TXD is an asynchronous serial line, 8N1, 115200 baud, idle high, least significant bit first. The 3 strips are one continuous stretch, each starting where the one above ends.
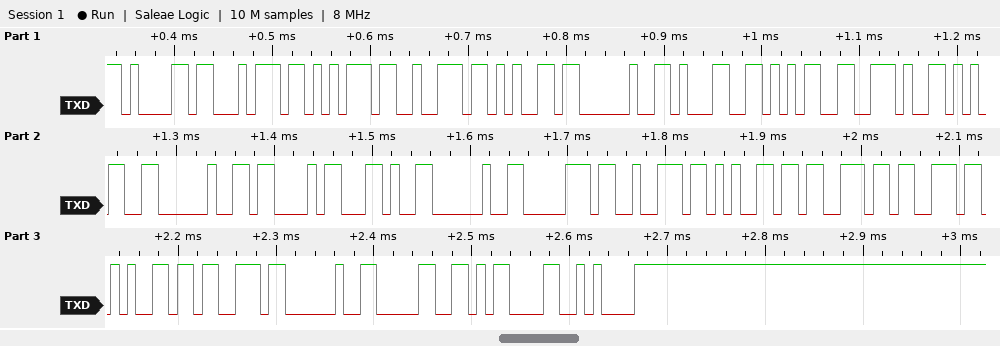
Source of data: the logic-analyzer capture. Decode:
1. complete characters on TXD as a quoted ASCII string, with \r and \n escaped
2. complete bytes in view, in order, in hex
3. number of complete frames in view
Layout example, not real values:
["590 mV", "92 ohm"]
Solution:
["\"ature 15.5 C, presses 0\\r\\n\"", "61 74 75 72 65 20 31 35 2E 35 20 43 2C 20 70 72 65 73 73 65 73 20 30 0D 0A", "25"]
